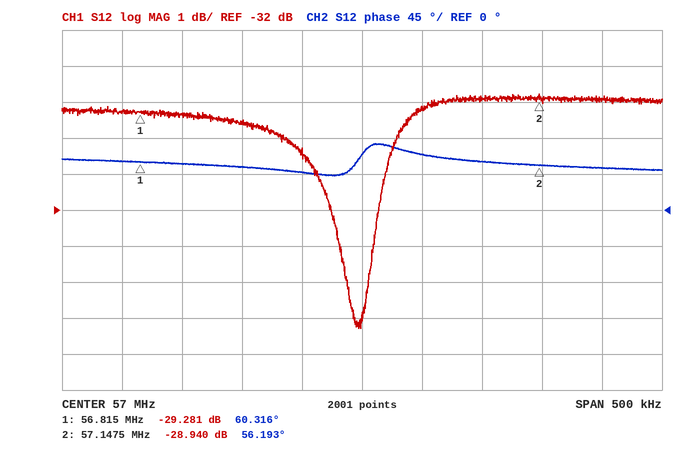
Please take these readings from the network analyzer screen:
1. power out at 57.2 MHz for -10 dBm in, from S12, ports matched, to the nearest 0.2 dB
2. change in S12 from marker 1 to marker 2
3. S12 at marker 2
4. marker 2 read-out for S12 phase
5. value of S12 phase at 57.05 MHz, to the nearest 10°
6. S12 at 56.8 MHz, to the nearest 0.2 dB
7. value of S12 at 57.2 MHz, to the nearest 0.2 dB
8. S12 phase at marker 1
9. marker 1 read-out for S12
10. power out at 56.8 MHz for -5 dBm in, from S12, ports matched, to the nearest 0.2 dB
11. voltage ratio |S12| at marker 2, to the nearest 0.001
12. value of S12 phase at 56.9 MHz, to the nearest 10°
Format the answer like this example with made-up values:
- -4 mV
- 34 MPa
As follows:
- -39.0 dBm
- 0.341 dB
- -28.940 dB
- 56.193°
- 70°
- -29.2 dB
- -29.0 dB
- 60.316°
- -29.281 dB
- -34.2 dBm
- 0.036
- 50°
